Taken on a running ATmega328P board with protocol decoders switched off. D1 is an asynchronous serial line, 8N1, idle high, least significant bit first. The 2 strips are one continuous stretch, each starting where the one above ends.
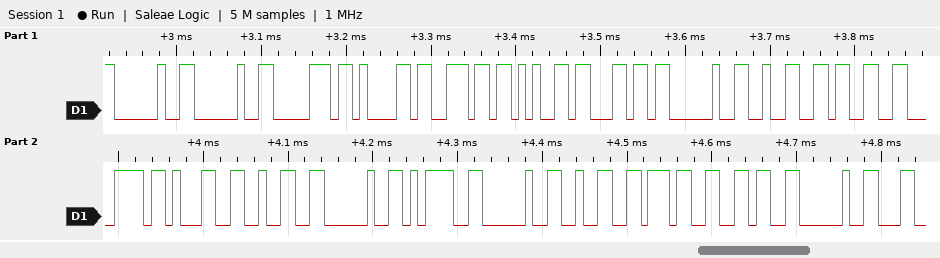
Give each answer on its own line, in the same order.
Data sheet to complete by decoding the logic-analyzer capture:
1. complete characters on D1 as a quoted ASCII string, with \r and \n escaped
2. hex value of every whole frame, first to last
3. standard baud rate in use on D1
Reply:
"  panel 23x12 = 276 "
20 20 70 61 6E 65 6C 20 32 33 78 31 32 20 3D 20 32 37 36 20
115200 baud
